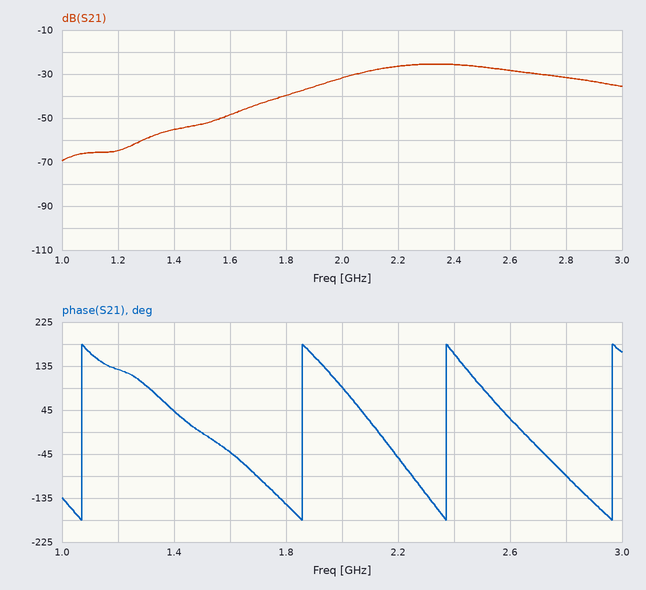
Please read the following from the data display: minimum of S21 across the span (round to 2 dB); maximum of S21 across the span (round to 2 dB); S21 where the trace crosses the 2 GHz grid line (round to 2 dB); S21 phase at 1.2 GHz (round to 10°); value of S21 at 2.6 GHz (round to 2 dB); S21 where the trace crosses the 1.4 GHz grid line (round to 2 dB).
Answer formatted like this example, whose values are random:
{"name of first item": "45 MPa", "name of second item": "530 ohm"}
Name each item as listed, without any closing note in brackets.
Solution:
{"minimum of S21 across the span": "-70 dB", "maximum of S21 across the span": "-26 dB", "S21 where the trace crosses the 2 GHz grid line": "-32 dB", "S21 phase at 1.2 GHz": "130°", "value of S21 at 2.6 GHz": "-28 dB", "S21 where the trace crosses the 1.4 GHz grid line": "-56 dB"}
